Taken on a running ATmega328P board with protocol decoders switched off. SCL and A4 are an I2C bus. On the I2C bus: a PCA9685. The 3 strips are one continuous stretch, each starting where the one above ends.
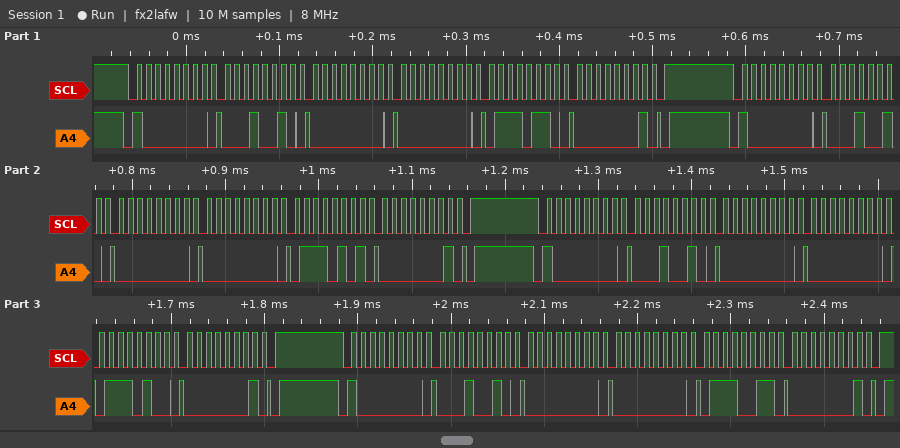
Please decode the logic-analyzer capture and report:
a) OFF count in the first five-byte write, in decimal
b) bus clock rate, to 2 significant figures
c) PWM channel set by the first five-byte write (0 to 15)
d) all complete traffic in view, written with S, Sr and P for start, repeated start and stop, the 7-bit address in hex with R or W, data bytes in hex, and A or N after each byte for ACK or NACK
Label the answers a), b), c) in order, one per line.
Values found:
a) 374
b) 100 kHz
c) 3
d) S 40W A 12 A 00 A 00 A 76 A 01 A P S 40W A 12 A 00 A 00 A 75 A 01 A P S 40W A 12 A 00 A 00 A 74 A 01 A P S 40W A 12 A 00 A 00 A 73 A 01 A P
